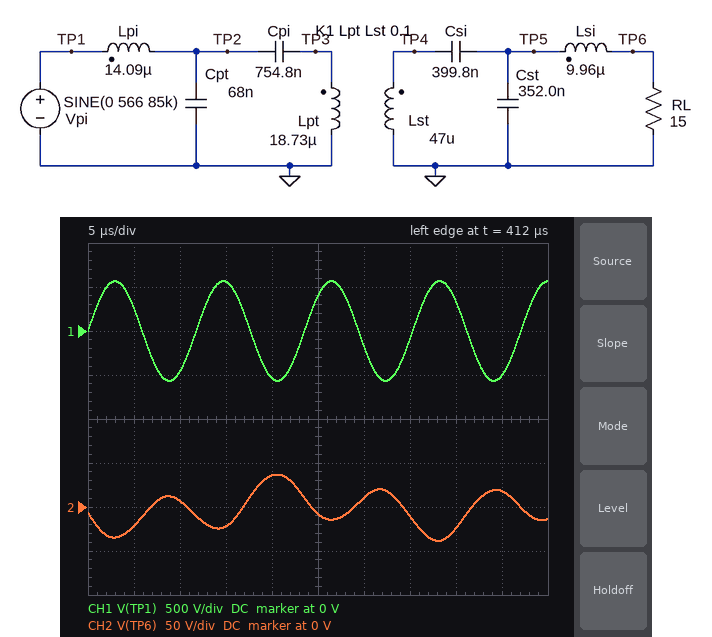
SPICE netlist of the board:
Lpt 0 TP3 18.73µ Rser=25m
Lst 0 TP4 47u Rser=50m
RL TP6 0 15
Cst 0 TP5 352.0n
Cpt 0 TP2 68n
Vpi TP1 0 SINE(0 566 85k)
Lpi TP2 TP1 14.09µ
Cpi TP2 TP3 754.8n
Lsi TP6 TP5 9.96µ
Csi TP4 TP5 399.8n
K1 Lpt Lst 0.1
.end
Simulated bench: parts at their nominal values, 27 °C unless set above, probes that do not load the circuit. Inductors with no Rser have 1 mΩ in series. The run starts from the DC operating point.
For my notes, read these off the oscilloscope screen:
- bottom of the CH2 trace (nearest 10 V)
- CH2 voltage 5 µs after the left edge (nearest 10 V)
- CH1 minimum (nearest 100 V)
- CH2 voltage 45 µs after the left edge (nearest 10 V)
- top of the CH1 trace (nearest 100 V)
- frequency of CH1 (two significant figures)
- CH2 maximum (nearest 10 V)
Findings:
-40 V
-20 V
-600 V
20 V
600 V
85 kHz
40 V
